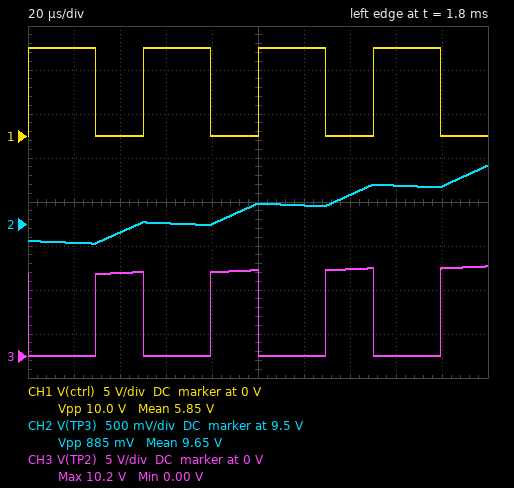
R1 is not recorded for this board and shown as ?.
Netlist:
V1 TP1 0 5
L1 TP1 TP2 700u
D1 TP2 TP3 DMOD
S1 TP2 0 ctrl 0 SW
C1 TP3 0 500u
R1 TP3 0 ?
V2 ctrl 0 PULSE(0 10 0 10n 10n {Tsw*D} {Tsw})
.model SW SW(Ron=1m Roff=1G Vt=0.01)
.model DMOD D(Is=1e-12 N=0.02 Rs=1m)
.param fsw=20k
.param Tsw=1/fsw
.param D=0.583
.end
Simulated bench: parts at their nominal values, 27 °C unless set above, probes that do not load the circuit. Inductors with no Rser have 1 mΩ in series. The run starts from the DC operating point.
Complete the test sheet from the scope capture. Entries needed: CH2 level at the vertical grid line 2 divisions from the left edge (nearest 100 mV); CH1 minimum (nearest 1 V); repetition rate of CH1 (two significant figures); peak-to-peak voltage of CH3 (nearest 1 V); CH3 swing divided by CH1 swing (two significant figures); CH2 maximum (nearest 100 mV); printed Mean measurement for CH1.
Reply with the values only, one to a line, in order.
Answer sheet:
9.4 V
0 V
20 kHz
10 V
1.0
10.2 V
5.85 V
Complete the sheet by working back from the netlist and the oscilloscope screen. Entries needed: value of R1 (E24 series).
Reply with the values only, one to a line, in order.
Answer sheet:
18 Ω
